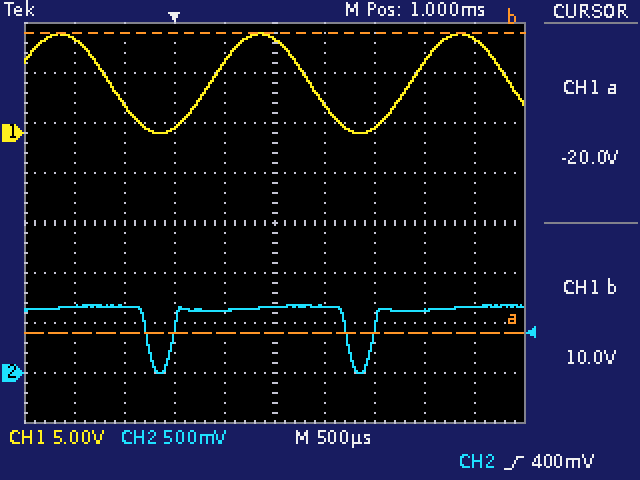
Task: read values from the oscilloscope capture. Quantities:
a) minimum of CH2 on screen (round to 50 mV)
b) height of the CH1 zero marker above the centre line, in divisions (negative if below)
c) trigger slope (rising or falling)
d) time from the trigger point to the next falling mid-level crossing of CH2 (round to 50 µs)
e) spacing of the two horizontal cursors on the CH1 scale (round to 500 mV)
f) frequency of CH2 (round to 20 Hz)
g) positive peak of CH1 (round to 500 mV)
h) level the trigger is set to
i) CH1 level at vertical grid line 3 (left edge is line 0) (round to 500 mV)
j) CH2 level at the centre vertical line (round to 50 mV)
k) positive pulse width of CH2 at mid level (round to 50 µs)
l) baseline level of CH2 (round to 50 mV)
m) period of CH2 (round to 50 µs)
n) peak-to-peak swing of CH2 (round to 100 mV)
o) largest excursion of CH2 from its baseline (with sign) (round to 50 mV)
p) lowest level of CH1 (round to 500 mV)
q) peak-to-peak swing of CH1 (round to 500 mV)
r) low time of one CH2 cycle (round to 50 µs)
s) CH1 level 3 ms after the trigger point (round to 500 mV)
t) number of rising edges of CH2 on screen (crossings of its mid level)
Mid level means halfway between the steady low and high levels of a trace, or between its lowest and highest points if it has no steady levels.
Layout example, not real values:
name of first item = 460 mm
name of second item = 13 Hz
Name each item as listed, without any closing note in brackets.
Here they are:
minimum of CH2 on screen = 0 mV
height of the CH1 zero marker above the centre line, in divisions = +1.8 div
trigger slope = rising
time from the trigger point to the next falling mid-level crossing of CH2 = 1.75 ms
spacing of the two horizontal cursors on the CH1 scale = 30.0 V
frequency of CH2 = 500 Hz
positive peak of CH1 = 10.0 V
level the trigger is set to = 400 mV
CH1 level at vertical grid line 3 (left edge is line 0) = 500 mV
CH2 level at the centre vertical line = 650 mV
positive pulse width of CH2 at mid level = 1.75 ms
baseline level of CH2 = 650 mV
period of CH2 = 2.00 ms
peak-to-peak swing of CH2 = 700 mV
largest excursion of CH2 from its baseline (with sign) = -650 mV
lowest level of CH1 = 0.0 V
peak-to-peak swing of CH1 = 10.0 V
low time of one CH2 cycle = 250 µs
CH1 level 3 ms after the trigger point = 9.5 V
number of rising edges of CH2 on screen = 2
